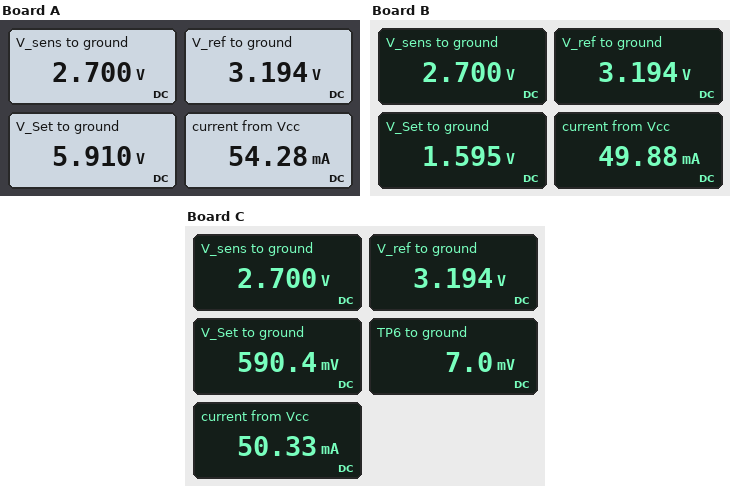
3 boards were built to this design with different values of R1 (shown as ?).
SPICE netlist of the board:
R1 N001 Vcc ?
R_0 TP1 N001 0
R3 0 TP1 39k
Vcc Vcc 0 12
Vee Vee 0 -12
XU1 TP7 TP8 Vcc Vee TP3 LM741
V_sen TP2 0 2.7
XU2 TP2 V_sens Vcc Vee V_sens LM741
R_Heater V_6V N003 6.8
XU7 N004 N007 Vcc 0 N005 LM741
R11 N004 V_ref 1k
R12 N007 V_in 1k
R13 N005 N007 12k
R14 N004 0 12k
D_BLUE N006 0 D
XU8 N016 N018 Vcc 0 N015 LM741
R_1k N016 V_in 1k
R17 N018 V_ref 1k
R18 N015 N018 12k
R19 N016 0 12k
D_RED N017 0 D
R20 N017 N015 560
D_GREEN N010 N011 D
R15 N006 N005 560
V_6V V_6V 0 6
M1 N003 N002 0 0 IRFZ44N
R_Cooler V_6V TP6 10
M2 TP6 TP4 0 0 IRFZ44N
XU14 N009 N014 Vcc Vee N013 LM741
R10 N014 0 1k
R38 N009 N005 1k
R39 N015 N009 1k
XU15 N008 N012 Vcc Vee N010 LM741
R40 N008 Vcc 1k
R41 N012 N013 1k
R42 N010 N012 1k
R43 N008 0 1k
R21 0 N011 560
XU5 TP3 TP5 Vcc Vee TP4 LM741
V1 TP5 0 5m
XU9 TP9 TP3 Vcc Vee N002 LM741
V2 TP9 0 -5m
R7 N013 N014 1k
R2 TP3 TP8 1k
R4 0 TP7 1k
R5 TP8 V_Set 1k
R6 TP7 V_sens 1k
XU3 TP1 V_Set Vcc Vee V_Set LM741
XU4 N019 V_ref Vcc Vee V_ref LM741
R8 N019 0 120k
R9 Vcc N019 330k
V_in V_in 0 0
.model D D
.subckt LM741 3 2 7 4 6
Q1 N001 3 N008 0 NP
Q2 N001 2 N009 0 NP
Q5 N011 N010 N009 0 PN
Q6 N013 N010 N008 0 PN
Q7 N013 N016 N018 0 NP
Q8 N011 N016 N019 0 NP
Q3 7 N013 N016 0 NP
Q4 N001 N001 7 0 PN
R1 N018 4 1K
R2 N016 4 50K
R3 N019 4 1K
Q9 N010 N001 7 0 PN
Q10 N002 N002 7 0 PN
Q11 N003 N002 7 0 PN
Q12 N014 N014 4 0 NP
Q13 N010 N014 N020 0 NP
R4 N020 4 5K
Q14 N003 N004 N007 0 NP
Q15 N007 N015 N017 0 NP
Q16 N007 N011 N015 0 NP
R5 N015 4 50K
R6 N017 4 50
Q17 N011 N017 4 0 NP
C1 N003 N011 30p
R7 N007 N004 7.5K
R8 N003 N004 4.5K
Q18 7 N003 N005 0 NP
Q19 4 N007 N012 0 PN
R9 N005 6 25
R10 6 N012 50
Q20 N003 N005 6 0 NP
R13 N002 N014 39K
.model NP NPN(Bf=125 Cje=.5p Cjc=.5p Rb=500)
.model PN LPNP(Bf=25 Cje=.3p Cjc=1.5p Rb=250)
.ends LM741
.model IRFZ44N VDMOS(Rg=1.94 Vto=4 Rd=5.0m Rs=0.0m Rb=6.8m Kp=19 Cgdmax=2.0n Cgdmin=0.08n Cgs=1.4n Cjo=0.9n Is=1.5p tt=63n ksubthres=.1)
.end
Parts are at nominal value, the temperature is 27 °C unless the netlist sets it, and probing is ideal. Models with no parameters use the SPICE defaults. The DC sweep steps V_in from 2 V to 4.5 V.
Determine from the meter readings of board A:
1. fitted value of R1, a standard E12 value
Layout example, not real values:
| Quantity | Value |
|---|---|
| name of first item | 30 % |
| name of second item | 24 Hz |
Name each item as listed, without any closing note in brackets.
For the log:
| Quantity | Value |
|---|---|
| fitted value of R1, a standard E12 value | 27 kΩ |
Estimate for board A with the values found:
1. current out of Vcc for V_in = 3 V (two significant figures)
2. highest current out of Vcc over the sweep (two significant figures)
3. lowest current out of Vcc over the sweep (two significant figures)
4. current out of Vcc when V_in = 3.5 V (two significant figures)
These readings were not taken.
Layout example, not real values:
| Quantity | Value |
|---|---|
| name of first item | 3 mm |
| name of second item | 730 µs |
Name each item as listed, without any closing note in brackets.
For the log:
| Quantity | Value |
|---|---|
| current out of Vcc for V_in = 3 V | 42 mA |
| highest current out of Vcc over the sweep | 54 mA |
| lowest current out of Vcc over the sweep | 42 mA |
| current out of Vcc when V_in = 3.5 V | 42 mA |
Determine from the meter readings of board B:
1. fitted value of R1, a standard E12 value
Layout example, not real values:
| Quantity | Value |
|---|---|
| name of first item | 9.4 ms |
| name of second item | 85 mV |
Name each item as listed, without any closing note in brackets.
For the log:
| Quantity | Value |
|---|---|
| fitted value of R1, a standard E12 value | 100 kΩ |
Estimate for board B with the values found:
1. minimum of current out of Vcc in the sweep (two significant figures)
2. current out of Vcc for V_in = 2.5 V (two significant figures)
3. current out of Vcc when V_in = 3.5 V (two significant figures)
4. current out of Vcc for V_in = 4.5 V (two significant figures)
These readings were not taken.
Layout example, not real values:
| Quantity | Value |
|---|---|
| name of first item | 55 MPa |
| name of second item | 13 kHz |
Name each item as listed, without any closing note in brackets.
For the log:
| Quantity | Value |
|---|---|
| minimum of current out of Vcc in the sweep | 37 mA |
| current out of Vcc for V_in = 2.5 V | 44 mA |
| current out of Vcc when V_in = 3.5 V | 38 mA |
| current out of Vcc for V_in = 4.5 V | 49 mA |
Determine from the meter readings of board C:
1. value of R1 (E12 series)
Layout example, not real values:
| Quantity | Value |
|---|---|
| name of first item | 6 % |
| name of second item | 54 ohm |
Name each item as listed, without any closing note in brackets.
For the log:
| Quantity | Value |
|---|---|
| value of R1 | 270 kΩ |
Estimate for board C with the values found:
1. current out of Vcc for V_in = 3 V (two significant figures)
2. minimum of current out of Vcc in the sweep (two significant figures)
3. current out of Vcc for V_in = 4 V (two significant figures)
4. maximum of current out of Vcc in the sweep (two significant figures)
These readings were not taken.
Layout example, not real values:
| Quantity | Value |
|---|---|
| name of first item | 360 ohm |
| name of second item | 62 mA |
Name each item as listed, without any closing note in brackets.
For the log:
| Quantity | Value |
|---|---|
| current out of Vcc for V_in = 3 V | 38 mA |
| minimum of current out of Vcc in the sweep | 38 mA |
| current out of Vcc for V_in = 4 V | 48 mA |
| maximum of current out of Vcc in the sweep | 50 mA |
